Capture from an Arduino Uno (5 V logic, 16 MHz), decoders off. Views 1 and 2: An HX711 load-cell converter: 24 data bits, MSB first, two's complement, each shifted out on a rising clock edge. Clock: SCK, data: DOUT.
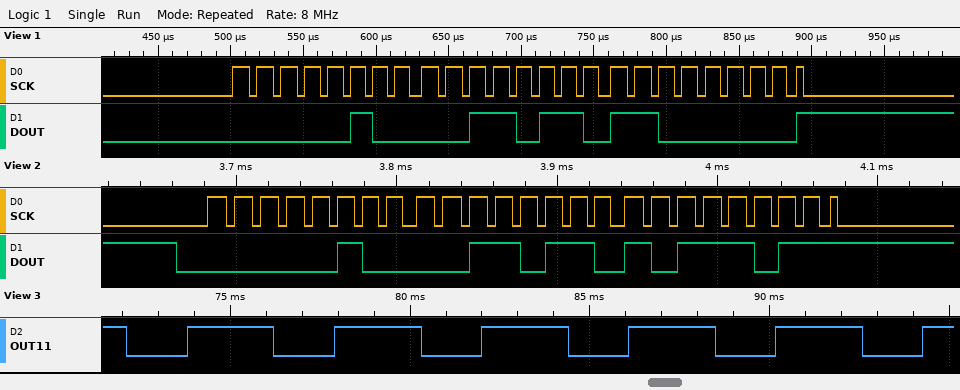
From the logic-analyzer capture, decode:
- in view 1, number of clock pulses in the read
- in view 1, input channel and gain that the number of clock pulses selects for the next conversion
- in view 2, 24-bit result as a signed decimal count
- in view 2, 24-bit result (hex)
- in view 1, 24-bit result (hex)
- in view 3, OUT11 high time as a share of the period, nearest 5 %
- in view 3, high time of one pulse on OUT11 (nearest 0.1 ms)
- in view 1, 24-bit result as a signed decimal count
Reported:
25
channel A, gain 128
276155
0x0436BB
0x0436C0
60 %
2.4 ms
276160
